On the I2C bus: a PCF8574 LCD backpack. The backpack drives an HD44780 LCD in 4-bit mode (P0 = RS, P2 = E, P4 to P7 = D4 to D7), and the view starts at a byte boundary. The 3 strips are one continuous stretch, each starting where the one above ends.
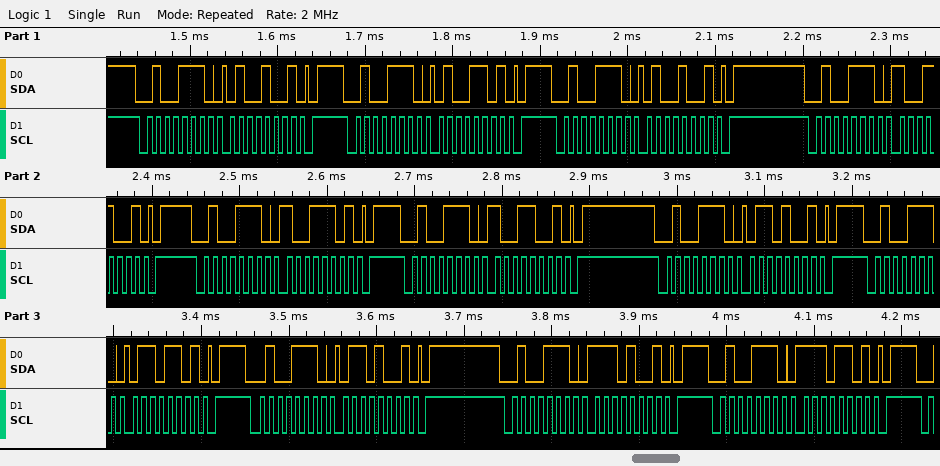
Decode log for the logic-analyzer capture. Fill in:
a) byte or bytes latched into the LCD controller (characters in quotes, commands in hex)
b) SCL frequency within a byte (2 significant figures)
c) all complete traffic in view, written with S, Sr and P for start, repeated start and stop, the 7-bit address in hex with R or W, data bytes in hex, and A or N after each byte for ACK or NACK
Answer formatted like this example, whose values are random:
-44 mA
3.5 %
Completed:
'I'
100 kHz
S 27W A 49 A P S 27W A 4D A P S 27W A 49 A P S 27W A 99 A P S 27W A 9D A P S 27W A 99 A P S 27W A 69 A P S 27W A 6D A P S 27W A 69 A P S 27W A E9 A P S 27W A ED A P
